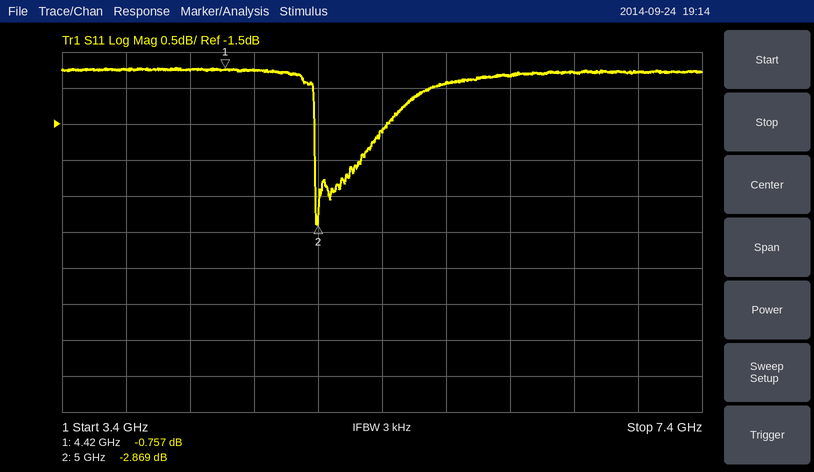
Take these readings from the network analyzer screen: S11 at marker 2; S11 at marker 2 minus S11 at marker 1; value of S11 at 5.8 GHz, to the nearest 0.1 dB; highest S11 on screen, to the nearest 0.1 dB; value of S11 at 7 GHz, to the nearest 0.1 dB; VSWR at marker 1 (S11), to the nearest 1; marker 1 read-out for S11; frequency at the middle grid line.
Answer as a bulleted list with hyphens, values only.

- -2.869 dB
- -2.112 dB
- -0.9 dB
- -0.7 dB
- -0.8 dB
- 23
- -0.757 dB
- 5.4 GHz
